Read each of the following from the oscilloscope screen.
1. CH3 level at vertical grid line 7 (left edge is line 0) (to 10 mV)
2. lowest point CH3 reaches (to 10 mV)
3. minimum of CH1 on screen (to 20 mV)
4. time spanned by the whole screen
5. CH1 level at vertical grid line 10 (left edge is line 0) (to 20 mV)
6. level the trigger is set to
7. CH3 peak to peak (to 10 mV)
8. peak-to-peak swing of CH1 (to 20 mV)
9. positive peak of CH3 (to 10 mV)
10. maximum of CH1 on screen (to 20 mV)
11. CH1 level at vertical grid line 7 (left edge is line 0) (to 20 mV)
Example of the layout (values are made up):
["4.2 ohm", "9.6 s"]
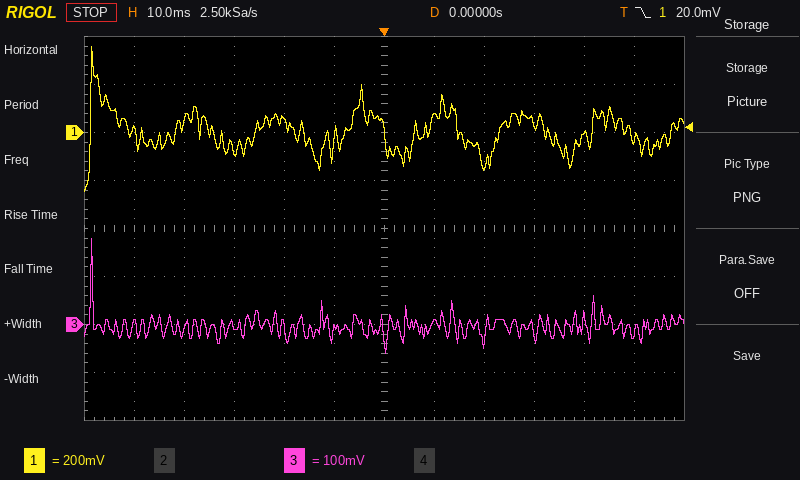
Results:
["0 mV", "-60 mV", "-240 mV", "120 ms", "0 mV", "20.0 mV", "240 mV", "600 mV", "180 mV", "360 mV", "60 mV"]
